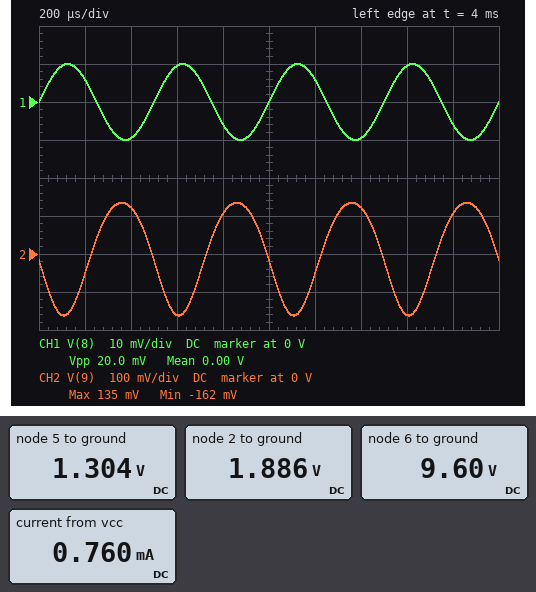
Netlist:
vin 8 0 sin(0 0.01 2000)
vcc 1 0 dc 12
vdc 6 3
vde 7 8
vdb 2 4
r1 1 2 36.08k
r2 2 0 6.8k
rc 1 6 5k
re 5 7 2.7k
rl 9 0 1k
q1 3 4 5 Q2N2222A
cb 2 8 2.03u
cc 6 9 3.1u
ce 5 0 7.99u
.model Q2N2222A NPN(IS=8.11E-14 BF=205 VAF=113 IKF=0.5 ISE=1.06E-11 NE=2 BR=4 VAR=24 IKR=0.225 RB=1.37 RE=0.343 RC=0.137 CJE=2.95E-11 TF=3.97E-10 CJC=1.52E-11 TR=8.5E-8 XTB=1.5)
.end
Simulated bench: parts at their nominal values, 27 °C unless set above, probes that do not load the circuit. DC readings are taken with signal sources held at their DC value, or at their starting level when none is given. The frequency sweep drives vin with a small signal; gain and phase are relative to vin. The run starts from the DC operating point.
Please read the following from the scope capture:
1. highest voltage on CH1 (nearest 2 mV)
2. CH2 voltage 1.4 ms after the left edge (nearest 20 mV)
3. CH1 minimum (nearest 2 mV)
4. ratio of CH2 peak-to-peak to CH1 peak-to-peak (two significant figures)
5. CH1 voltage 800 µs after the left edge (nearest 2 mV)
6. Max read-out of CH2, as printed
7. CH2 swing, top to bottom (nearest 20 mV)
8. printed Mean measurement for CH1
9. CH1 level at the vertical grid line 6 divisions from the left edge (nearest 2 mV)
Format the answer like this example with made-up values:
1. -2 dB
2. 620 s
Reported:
1. 10 mV
2. 120 mV
3. -10 mV
4. 15
5. -6 mV
6. 135 mV
7. 300 mV
8. 0.00 V
9. 6 mV
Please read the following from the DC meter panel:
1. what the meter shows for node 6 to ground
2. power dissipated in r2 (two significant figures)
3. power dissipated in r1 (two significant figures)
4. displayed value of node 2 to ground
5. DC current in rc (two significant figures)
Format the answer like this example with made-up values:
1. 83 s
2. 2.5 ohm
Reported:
1. 9.60 V
2. 520 µW
3. 2.8 mW
4. 1.886 V
5. 480 µA
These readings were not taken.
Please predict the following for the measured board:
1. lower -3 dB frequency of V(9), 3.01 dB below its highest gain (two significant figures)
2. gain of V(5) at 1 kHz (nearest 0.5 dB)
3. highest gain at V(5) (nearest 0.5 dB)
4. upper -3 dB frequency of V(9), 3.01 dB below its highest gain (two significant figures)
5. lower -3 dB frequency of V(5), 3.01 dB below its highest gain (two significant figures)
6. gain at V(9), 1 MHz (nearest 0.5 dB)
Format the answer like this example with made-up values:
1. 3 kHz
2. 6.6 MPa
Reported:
1. 380 Hz
2. -9.0 dB
3. -0.5 dB
4. 27 MHz
5. 13 Hz
6. 23.5 dB
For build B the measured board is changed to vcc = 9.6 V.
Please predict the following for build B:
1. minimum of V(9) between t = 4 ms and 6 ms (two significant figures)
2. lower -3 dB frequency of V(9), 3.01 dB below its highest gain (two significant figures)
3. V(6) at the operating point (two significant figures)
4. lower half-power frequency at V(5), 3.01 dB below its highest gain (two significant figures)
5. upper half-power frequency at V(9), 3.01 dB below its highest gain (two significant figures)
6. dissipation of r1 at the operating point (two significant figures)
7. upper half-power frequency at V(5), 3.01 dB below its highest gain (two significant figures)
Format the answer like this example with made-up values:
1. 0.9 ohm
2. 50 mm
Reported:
1. -120 mV
2. 280 Hz
3. 7.9 V
4. 12 Hz
5. 26 MHz
6. 1.8 mW
7. 300 Hz
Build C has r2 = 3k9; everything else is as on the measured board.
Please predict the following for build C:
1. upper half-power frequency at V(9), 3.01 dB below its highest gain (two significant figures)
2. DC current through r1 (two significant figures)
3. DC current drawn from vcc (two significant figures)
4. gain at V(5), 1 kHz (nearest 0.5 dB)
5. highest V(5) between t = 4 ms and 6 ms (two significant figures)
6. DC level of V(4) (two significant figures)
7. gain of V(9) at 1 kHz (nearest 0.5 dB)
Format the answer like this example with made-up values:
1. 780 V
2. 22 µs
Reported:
1. 30 MHz
2. 300 µA
3. 520 µA
4. -15.0 dB
5. 610 mV
6. 1.2 V
7. 17.0 dB
